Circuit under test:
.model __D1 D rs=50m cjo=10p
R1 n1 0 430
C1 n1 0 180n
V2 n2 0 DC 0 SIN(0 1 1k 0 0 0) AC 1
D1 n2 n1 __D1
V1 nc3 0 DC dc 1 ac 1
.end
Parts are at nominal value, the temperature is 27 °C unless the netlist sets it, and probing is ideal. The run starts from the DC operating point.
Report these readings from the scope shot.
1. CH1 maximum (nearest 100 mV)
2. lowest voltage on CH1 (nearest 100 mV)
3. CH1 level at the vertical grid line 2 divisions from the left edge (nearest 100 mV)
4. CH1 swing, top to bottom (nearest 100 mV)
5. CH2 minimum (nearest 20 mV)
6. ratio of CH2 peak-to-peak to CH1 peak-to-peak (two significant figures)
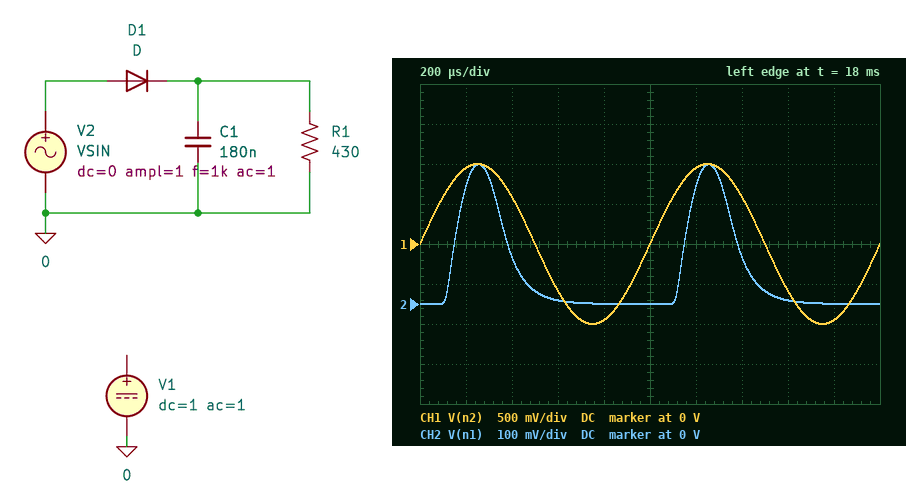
1.0 V
-1.0 V
600 mV
2.0 V
0 V
0.17
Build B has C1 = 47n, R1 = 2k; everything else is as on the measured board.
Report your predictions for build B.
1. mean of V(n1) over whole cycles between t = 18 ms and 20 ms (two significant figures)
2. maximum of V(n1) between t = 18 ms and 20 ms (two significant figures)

95 mV
390 mV
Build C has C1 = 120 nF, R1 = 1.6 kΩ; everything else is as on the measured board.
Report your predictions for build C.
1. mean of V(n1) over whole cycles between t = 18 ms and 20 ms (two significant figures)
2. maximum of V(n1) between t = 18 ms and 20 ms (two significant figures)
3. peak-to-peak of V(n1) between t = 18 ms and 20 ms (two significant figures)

120 mV
380 mV
370 mV
